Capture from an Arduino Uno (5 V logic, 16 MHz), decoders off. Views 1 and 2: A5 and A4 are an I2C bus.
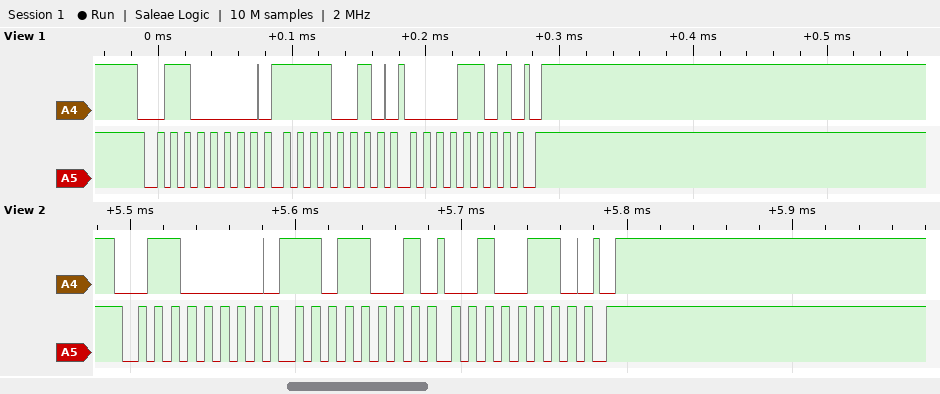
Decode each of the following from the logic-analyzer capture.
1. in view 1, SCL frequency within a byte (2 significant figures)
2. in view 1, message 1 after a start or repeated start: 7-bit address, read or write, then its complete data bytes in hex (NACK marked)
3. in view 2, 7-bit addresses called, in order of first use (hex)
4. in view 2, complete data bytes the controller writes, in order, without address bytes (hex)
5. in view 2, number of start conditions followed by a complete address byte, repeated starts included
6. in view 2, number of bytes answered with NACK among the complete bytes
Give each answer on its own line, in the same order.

100 kHz
0x30 write: F2 0D
0x30
D9 26
1
0
